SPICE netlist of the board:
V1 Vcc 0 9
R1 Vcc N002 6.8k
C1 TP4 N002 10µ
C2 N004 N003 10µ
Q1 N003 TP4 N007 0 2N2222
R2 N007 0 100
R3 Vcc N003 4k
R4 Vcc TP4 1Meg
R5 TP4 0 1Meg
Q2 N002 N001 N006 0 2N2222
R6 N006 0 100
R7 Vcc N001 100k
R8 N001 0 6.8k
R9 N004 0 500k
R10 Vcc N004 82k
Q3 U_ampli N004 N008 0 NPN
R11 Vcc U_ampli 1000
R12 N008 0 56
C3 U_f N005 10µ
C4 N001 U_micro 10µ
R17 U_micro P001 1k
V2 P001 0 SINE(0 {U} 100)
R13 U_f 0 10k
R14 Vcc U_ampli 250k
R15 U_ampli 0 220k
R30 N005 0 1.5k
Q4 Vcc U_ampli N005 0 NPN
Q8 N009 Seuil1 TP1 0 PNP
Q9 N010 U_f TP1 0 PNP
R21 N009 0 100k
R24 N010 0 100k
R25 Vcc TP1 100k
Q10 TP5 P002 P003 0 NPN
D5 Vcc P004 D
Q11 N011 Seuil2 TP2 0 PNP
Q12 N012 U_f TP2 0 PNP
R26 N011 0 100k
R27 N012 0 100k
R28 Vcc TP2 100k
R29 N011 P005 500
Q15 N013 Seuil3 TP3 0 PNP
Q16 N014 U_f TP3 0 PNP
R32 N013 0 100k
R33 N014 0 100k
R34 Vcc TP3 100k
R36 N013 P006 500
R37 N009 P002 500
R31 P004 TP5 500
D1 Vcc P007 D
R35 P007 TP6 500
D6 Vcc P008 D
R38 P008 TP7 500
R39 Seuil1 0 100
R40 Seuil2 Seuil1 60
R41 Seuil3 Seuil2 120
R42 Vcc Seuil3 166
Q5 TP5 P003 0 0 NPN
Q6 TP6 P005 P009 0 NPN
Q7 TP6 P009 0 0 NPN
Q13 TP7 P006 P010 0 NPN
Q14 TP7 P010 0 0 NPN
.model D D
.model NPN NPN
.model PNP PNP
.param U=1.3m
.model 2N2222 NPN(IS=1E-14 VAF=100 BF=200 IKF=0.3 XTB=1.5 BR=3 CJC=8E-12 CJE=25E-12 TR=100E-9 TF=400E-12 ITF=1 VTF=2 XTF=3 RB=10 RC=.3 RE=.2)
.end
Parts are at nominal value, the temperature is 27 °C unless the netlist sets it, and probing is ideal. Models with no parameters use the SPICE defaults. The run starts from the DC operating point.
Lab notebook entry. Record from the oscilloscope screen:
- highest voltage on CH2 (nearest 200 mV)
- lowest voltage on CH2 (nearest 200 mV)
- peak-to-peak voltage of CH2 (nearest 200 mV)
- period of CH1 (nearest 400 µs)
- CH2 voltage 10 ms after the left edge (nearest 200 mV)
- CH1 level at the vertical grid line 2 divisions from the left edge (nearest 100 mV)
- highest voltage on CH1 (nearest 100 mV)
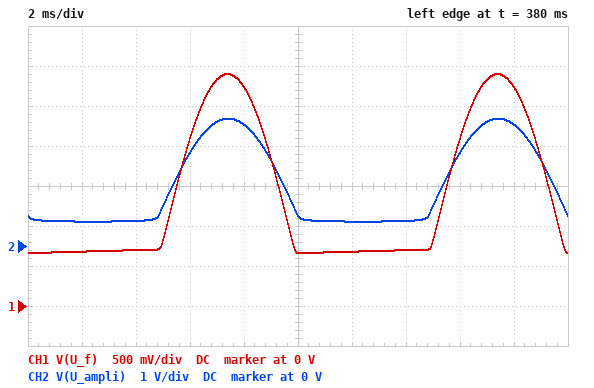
3.2 V
600 mV
2.6 V
10.0 ms
800 mV
700 mV
2.9 V
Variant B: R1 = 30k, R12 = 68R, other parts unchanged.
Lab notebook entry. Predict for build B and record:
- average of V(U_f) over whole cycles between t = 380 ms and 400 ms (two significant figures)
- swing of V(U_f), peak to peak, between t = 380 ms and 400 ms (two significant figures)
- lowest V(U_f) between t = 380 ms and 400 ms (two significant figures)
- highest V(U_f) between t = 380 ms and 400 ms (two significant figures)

1.5 V
5.6 V
-480 mV
5.1 V
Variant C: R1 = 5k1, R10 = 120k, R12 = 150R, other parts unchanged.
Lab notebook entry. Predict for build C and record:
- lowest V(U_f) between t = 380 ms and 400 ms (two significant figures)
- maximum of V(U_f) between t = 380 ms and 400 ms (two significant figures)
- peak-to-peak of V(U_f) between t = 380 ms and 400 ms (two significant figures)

420 mV
2.3 V
1.9 V
